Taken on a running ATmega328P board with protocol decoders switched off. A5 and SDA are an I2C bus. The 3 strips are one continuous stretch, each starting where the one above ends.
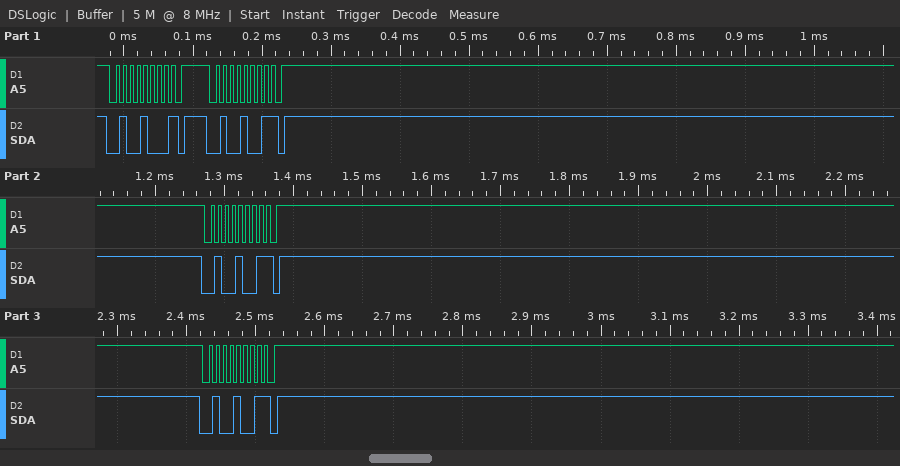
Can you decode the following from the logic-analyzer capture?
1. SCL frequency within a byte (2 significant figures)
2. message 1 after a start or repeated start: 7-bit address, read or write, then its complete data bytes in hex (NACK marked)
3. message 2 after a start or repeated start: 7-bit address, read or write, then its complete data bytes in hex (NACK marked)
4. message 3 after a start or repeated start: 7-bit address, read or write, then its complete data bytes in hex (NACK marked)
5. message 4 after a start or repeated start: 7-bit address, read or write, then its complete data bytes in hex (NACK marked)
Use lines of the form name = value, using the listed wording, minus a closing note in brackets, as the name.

SCL frequency within a byte = 100 kHz
message 1 after a start or repeated start: 7-bit address, read or write, then its complete data bytes in hex = 0x24 write NACK
message 2 after a start or repeated start: 7-bit address, read or write, then its complete data bytes in hex = 0x24 read NACK
message 3 after a start or repeated start: 7-bit address, read or write, then its complete data bytes in hex = 0x24 read NACK
message 4 after a start or repeated start: 7-bit address, read or write, then its complete data bytes in hex = 0x24 read NACK
